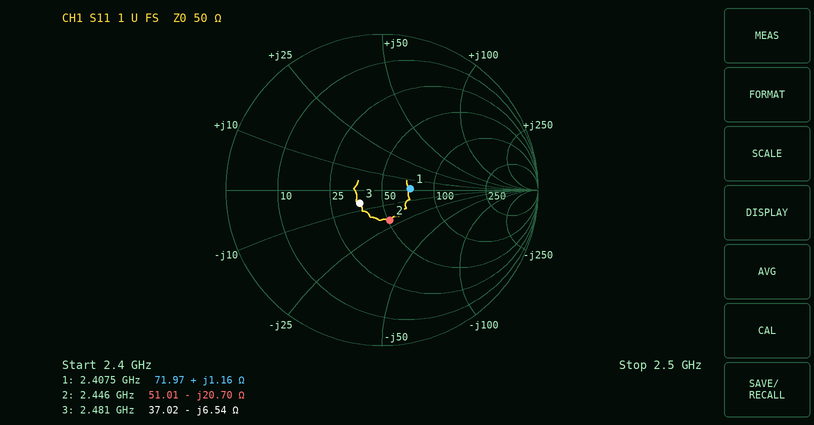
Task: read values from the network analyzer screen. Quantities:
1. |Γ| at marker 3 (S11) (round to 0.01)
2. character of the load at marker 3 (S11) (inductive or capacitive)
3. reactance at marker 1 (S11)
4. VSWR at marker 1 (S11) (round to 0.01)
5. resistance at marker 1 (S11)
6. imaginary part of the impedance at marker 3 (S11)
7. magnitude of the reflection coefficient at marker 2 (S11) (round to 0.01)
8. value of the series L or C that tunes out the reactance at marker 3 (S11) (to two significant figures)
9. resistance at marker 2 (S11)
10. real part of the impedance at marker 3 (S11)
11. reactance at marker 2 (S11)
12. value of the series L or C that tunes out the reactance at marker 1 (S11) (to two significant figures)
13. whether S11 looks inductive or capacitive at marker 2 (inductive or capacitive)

0.17
capacitive
+1.16 Ω
1.44
71.97 Ω
-6.54 Ω
0.20
420 pH
51.01 Ω
37.02 Ω
-20.70 Ω
57 pF
capacitive
